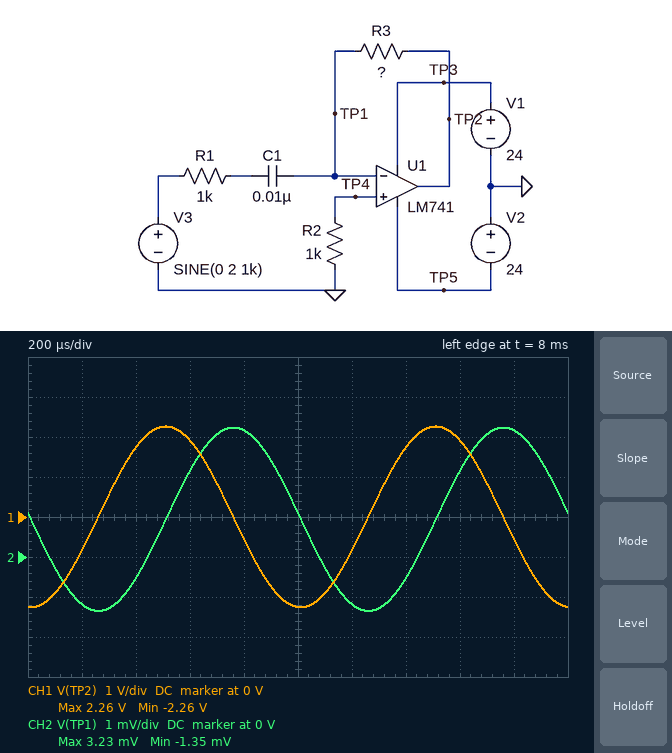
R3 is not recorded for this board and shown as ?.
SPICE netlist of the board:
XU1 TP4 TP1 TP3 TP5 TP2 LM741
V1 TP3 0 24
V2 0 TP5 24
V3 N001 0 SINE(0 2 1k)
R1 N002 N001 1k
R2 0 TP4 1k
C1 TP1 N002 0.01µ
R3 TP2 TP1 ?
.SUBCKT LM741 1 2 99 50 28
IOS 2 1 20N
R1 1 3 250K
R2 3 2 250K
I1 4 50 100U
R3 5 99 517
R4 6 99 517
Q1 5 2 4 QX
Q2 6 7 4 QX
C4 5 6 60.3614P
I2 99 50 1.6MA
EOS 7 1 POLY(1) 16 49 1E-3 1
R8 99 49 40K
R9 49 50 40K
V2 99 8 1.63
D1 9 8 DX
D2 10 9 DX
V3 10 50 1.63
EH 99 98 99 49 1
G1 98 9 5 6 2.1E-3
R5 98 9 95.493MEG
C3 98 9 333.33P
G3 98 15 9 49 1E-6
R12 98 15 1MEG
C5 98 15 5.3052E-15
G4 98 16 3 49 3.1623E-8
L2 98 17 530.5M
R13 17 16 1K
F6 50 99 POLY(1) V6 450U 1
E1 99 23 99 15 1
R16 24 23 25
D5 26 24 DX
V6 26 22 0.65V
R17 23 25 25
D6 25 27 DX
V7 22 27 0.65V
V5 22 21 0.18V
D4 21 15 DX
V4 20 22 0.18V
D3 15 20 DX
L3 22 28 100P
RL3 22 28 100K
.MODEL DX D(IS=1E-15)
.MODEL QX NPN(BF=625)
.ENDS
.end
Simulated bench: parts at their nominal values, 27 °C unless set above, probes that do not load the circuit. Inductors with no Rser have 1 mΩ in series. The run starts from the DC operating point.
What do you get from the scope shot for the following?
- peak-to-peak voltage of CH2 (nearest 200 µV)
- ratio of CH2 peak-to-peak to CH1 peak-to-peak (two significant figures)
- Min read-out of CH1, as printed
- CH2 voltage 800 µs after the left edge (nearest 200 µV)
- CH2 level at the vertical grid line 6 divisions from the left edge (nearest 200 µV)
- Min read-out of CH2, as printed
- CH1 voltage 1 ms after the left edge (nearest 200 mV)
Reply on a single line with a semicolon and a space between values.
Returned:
4.6 mV; 0.0010; -2.26 V; 3.2 mV; -1.2 mV; -1.35 mV; -2.2 V
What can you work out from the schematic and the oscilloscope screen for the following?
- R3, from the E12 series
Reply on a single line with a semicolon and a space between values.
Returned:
18 kΩ
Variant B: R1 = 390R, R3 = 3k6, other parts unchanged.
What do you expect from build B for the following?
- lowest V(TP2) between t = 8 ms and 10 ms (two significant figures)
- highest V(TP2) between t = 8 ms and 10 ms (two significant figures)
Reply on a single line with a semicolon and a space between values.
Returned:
-450 mV; 450 mV
